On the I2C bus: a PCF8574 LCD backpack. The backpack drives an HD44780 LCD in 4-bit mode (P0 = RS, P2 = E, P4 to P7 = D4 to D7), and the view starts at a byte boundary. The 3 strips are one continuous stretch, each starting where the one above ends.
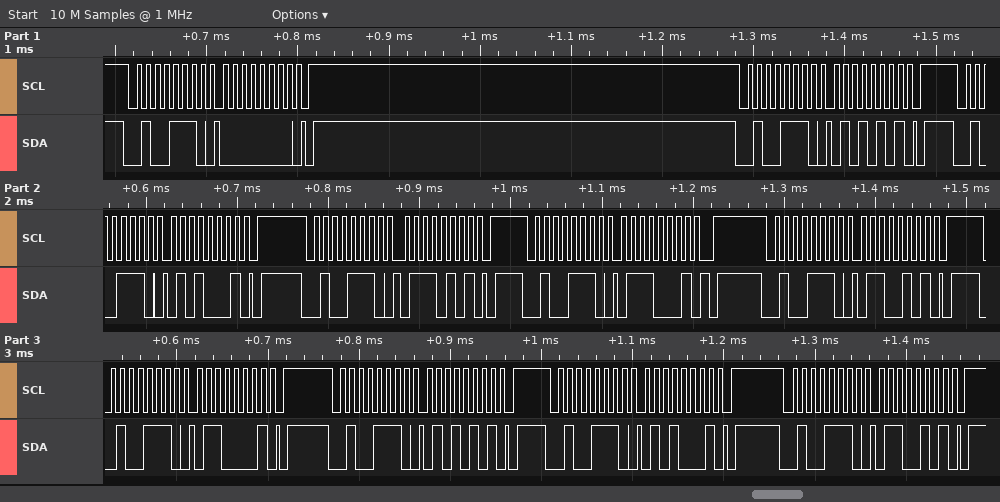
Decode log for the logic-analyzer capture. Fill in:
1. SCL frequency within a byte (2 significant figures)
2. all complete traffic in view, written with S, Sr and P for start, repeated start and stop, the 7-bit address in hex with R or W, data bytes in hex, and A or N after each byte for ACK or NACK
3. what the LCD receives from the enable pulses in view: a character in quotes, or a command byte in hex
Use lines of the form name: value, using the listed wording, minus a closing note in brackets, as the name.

SCL frequency within a byte: 100 kHz
all complete traffic in view, written with S, Sr and P for start, repeated start and stop, the 7-bit address in hex with R or W, data bytes in hex, and A or N after each byte for ACK or NACK: S 27W A 00 A P S 27W A 55 A P S 27W A 51 A P S 27W A 75 A P S 27W A 71 A P S 27W A 65 A P S 27W A 61 A P S 27W A 55 A P S 27W A 51 A P S 27W A 65 A P
what the LCD receives from the enable pulses in view: a character in quotes, or a command byte in hex: 'W' 'e'
